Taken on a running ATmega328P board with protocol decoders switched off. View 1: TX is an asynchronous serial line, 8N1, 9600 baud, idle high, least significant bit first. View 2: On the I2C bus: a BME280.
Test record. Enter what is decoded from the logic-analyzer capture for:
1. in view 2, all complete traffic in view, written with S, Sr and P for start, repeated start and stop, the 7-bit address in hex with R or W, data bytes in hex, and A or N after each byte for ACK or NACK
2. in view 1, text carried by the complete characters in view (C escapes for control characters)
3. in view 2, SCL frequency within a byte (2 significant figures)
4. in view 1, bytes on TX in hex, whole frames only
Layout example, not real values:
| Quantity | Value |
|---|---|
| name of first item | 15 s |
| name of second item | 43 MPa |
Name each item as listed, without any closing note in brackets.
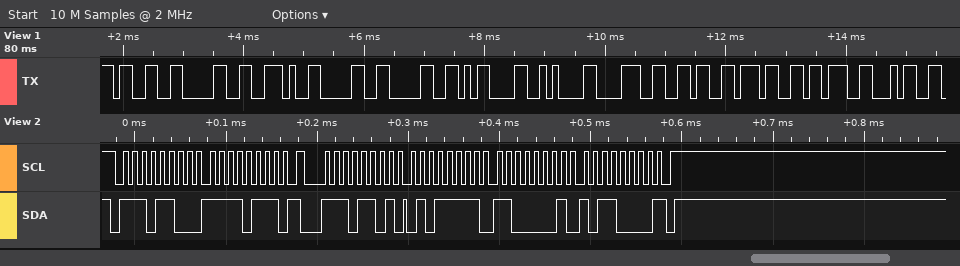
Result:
| Quantity | Value |
|---|---|
| in view 2, all complete traffic in view, written with S, Sr and P for start, repeated start and stop, the 7-bit address in hex with R or W, data bytes in hex, and A or N after each byte for ACK or NACK | S 76W A F7 A Sr 76R A 5F A C1 A B0 N P |
| in view 1, text carried by the complete characters in view | "30.00\r\n867;4" |
| in view 2, SCL frequency within a byte | 100 kHz |
| in view 1, bytes on TX in hex, whole frames only | 33 30 2E 30 30 0D 0A 38 36 37 3B 34 |
